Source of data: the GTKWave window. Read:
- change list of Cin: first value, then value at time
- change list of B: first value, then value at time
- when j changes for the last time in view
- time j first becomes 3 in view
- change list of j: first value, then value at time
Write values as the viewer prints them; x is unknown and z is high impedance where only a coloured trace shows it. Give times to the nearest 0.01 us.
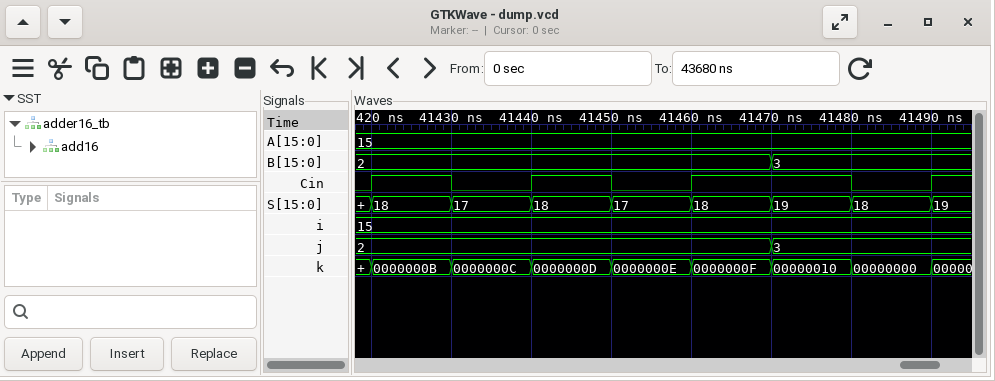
0, 1 at 41.42 us, 0 at 41.43 us, 1 at 41.44 us, 0 at 41.45 us, 1 at 41.46 us, 0 at 41.48 us, 1 at 41.49 us
2, 3 at 41.47 us
41.47 us
41.47 us
2, 3 at 41.47 us
